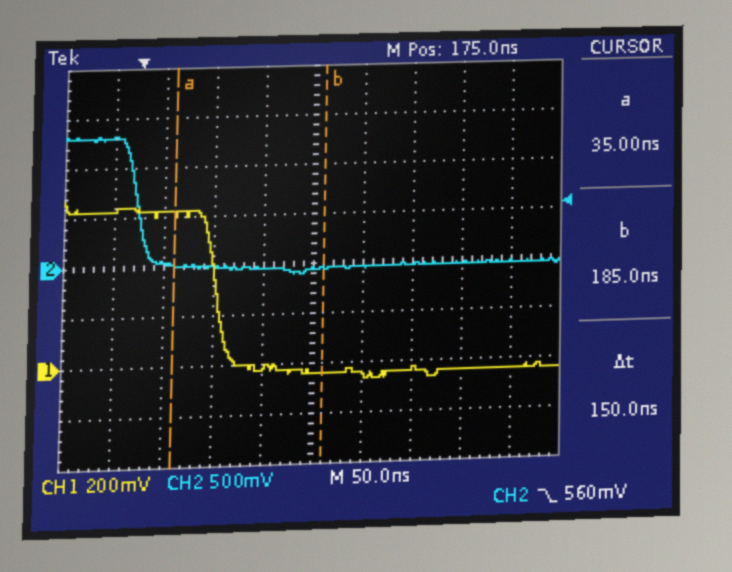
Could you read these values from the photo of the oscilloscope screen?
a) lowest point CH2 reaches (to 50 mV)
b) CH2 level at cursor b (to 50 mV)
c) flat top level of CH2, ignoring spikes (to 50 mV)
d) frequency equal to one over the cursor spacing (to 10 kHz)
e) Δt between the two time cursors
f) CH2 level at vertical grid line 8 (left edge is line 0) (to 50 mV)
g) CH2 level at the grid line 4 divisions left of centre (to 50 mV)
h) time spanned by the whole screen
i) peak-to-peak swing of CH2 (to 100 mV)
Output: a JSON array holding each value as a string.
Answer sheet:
["-100 mV", "-50 mV", "1.30 V", "6.67 MHz", "150 ns", "-50 mV", "1.30 V", "500 ns", "1.40 V"]
